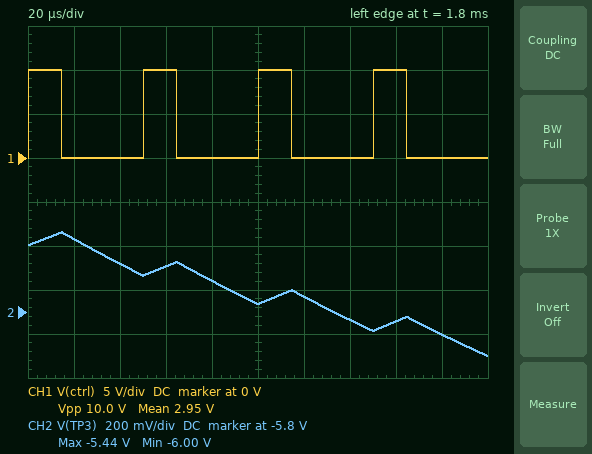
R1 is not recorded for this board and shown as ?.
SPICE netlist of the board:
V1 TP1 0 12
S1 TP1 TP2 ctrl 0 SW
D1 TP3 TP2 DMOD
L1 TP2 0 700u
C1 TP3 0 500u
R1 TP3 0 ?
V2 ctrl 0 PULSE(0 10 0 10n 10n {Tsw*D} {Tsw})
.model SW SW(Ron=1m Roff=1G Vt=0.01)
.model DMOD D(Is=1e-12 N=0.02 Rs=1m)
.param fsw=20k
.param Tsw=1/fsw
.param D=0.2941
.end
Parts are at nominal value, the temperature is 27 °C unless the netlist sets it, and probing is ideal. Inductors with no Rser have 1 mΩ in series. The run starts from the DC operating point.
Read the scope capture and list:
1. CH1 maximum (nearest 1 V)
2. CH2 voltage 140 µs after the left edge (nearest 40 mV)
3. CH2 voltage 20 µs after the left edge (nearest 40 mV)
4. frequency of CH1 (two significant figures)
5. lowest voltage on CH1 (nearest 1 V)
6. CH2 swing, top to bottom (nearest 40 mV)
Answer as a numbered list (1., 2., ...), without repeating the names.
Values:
1. 10 V
2. -5.84 V
3. -5.48 V
4. 20 kHz
5. 0 V
6. 560 mV
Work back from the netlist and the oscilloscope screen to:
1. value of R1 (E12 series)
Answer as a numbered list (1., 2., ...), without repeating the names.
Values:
1. 2.7 Ω
